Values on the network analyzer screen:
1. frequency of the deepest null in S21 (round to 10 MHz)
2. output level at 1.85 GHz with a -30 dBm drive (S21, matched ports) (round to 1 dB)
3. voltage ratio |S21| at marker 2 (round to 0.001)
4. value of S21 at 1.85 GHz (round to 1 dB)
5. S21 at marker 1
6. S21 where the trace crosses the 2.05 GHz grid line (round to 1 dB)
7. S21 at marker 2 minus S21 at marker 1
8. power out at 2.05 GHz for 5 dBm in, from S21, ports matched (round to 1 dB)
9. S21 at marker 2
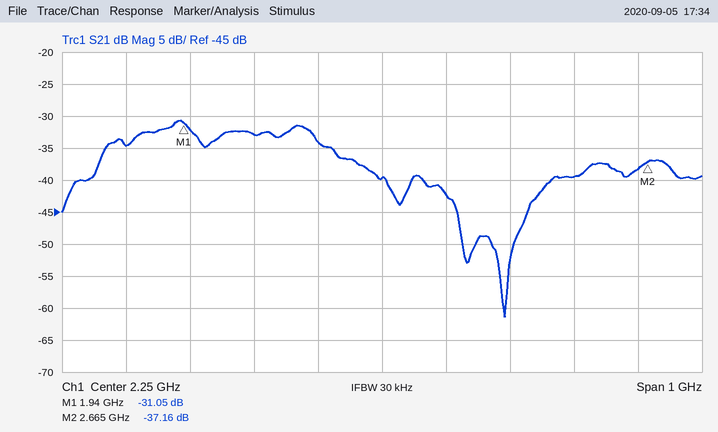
2.44 GHz
-65 dBm
0.014
-35 dB
-31.05 dB
-33 dB
-6.11 dB
-28 dBm
-37.16 dB
